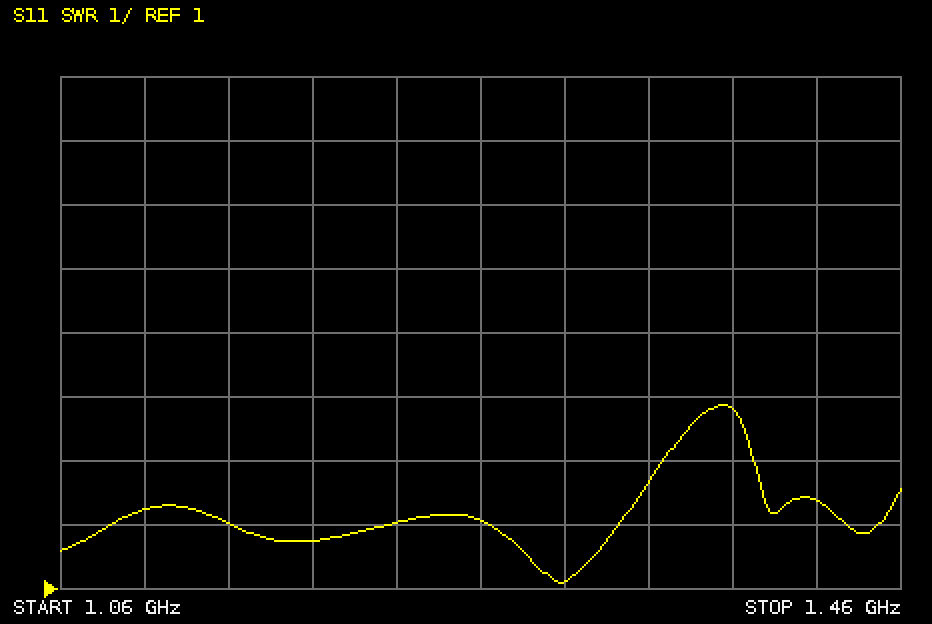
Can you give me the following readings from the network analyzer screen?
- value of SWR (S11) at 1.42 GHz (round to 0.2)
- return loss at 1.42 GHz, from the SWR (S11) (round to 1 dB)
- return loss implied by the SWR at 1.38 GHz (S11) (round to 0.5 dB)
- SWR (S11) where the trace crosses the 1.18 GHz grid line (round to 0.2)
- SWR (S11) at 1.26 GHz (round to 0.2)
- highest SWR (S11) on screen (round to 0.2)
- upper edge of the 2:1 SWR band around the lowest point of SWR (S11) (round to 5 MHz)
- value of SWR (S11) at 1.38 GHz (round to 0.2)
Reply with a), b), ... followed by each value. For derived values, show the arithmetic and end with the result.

a) 2.4
b) −20 log10((2.4 − 1)/(2.4 + 1)) ≈ 8 dB
c) −20 log10((3.8 − 1)/(3.8 + 1)) ≈ 4.68 dB, so 4.5 dB to the nearest 0.5 dB
d) 1.8
e) 2.0
f) 3.8
g) 1.325 GHz
h) 3.8
